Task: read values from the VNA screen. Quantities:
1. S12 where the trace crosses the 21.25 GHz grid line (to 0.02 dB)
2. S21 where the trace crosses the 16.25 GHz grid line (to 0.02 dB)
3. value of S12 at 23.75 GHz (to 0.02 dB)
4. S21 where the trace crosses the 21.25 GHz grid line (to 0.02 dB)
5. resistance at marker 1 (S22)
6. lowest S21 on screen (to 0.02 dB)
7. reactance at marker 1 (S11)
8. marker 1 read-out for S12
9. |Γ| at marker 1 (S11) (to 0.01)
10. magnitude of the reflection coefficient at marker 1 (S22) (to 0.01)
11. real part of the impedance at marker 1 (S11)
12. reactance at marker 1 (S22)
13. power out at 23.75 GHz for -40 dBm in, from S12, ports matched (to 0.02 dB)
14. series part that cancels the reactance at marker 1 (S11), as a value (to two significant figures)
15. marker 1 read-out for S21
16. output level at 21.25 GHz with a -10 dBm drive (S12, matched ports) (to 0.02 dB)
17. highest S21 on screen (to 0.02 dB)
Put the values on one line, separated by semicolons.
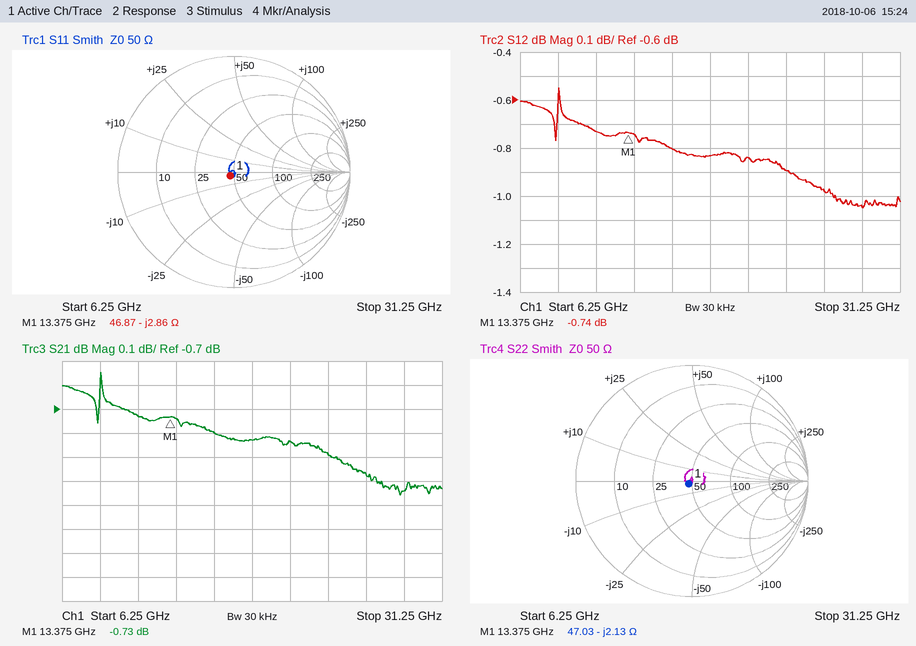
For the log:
-0.84 dB; -0.80 dB; -0.90 dB; -0.84 dB; 47.03 Ω; -1.06 dB; -2.86 Ω; -0.74 dB; 0.04; 0.04; 46.87 Ω; -2.13 Ω; -40.90 dBm; 34 pH; -0.73 dB; -10.84 dBm; -0.54 dB
